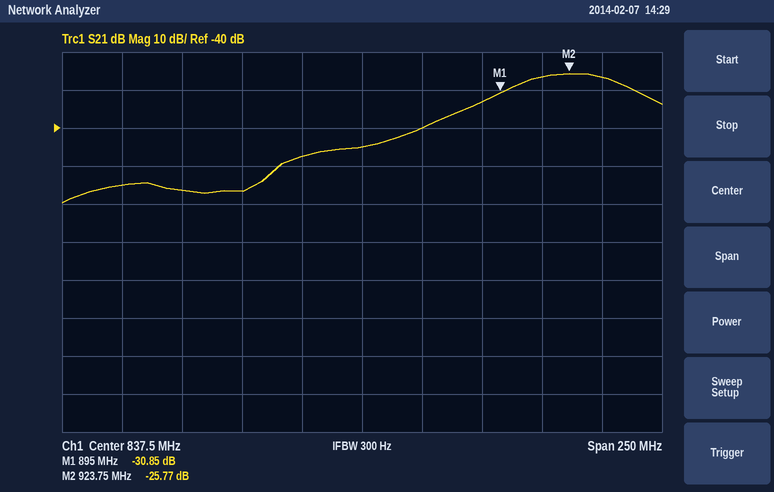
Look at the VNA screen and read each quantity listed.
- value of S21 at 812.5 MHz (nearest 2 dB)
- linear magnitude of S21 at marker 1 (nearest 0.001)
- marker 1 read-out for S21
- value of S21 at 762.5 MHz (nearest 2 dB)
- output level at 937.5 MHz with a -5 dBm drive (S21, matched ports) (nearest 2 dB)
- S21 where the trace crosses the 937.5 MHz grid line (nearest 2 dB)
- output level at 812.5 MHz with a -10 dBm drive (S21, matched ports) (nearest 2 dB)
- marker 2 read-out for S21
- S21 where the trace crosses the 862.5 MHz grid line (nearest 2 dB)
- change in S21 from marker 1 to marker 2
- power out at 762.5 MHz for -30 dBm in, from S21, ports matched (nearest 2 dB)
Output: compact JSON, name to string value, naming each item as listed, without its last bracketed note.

{"value of S21 at 812.5 MHz": "-48 dB", "linear magnitude of S21 at marker 1": "0.029", "marker 1 read-out for S21": "-30.85 dB", "value of S21 at 762.5 MHz": "-56 dB", "output level at 937.5 MHz with a -5 dBm drive (S21, matched ports)": "-32 dBm", "S21 where the trace crosses the 937.5 MHz grid line": "-26 dB", "output level at 812.5 MHz with a -10 dBm drive (S21, matched ports)": "-58 dBm", "marker 2 read-out for S21": "-25.77 dB", "S21 where the trace crosses the 862.5 MHz grid line": "-40 dB", "change in S21 from marker 1 to marker 2": "5.08 dB", "power out at 762.5 MHz for -30 dBm in, from S21, ports matched": "-86 dBm"}
